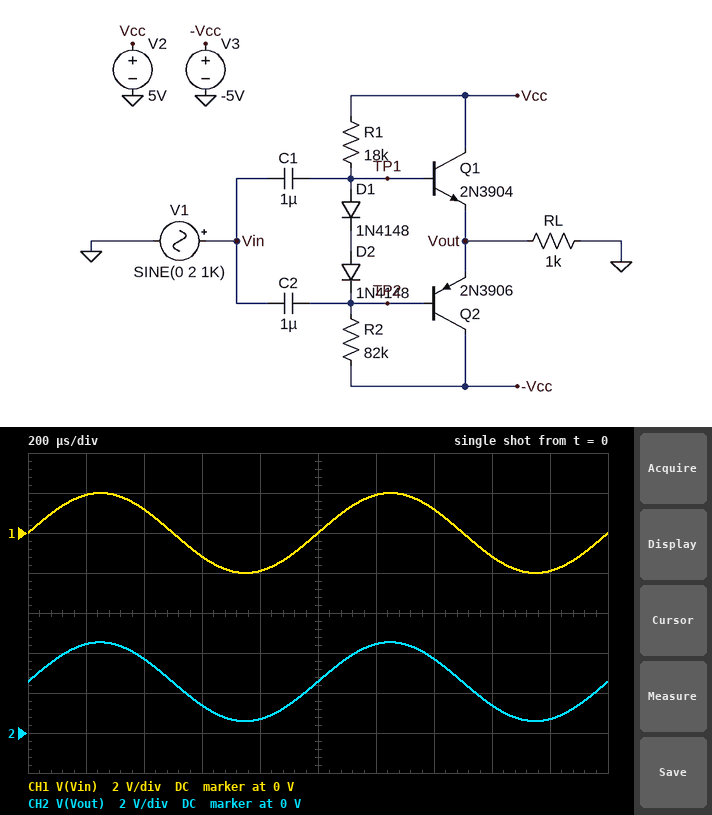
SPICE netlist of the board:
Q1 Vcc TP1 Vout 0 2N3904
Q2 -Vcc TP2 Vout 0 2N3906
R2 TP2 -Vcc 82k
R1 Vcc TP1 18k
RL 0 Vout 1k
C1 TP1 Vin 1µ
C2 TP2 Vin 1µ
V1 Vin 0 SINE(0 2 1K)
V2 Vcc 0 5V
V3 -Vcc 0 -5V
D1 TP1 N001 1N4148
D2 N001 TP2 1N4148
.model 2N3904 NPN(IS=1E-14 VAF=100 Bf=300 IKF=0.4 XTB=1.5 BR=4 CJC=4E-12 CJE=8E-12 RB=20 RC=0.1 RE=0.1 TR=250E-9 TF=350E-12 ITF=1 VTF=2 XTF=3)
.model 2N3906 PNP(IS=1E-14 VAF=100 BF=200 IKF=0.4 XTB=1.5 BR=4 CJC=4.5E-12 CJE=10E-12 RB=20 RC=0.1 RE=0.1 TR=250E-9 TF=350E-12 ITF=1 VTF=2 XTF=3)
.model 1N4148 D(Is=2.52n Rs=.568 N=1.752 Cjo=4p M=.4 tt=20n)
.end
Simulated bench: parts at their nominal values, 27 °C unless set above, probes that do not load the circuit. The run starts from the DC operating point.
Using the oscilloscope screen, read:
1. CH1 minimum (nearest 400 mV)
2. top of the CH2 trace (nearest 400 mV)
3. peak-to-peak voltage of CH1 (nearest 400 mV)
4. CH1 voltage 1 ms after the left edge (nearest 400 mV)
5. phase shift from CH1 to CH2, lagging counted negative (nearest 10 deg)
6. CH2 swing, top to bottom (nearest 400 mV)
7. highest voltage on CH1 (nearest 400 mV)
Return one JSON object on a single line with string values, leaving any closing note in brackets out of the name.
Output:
{"CH1 minimum": "-2.0 V", "top of the CH2 trace": "4.4 V", "peak-to-peak voltage of CH1": "4.0 V", "CH1 voltage 1 ms after the left edge": "0 V", "phase shift from CH1 to CH2, lagging counted negative": "0 deg", "CH2 swing, top to bottom": "4.0 V", "highest voltage on CH1": "2.0 V"}
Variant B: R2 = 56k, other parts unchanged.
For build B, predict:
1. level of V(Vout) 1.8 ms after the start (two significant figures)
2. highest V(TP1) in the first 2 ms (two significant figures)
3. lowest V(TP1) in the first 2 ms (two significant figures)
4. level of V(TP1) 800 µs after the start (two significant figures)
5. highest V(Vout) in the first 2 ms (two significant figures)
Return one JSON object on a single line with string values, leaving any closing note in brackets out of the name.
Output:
{"level of V(Vout) 1.8 ms after the start": "200 mV", "highest V(TP1) in the first 2 ms": "4.7 V", "lowest V(TP1) in the first 2 ms": "700 mV", "level of V(TP1) 800 µs after the start": "810 mV", "highest V(Vout) in the first 2 ms": "4.0 V"}
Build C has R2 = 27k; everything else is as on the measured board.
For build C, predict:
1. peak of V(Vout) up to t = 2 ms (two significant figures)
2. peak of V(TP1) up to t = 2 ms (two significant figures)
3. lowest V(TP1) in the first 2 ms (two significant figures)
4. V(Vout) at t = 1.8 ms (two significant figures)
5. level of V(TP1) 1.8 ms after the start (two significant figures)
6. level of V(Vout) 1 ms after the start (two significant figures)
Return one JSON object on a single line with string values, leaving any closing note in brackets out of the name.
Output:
{"peak of V(Vout) up to t = 2 ms": "2.7 V", "peak of V(TP1) up to t = 2 ms": "3.4 V", "lowest V(TP1) in the first 2 ms": "-630 mV", "V(Vout) at t = 1.8 ms": "-900 mV", "level of V(TP1) 1.8 ms after the start": "-530 mV", "level of V(Vout) 1 ms after the start": "740 mV"}
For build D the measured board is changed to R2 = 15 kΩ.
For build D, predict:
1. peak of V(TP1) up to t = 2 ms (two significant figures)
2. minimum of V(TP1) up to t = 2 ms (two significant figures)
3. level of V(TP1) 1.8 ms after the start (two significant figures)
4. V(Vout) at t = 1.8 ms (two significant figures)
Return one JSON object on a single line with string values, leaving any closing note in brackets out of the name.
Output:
{"peak of V(TP1) up to t = 2 ms": "2.1 V", "minimum of V(TP1) up to t = 2 ms": "-1.9 V", "level of V(TP1) 1.8 ms after the start": "-1.8 V", "V(Vout) at t = 1.8 ms": "-2.2 V"}
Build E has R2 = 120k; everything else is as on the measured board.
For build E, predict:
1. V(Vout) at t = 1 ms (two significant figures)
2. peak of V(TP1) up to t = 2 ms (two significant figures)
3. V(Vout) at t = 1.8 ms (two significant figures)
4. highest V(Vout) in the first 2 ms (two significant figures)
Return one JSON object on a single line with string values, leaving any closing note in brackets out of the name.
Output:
{"V(Vout) at t = 1 ms": "3.0 V", "peak of V(TP1) up to t = 2 ms": "5.6 V", "V(Vout) at t = 1.8 ms": "1.1 V", "highest V(Vout) in the first 2 ms": "4.9 V"}
